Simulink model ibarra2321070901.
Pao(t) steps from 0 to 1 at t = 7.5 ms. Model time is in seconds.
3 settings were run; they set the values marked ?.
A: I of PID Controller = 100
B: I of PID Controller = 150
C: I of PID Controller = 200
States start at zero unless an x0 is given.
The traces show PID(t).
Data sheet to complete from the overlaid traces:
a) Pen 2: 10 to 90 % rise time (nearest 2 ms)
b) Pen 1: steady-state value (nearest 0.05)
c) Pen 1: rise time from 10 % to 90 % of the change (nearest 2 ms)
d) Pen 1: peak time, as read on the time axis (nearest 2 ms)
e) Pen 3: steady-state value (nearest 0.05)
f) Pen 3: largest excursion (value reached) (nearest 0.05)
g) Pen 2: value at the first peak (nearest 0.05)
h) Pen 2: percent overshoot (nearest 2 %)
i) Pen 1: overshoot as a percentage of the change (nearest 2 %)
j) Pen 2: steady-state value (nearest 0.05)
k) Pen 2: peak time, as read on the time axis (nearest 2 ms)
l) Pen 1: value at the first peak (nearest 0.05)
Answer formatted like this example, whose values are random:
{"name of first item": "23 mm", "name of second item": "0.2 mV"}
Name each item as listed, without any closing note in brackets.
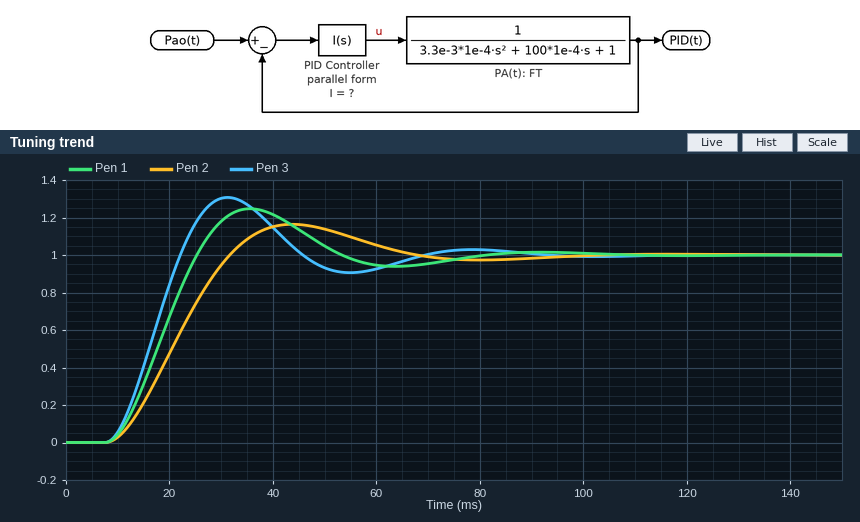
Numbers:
{"Pen 2: 10 to 90 % rise time": "16 ms", "Pen 1: steady-state value": "1.00", "Pen 1: rise time from 10 % to 90 % of the change": "12 ms", "Pen 1: peak time, as read on the time axis": "36 ms", "Pen 3: steady-state value": "1.00", "Pen 3: largest excursion (value reached)": "1.30", "Pen 2: value at the first peak": "1.15", "Pen 2: percent overshoot": "16 %", "Pen 1: overshoot as a percentage of the change": "24 %", "Pen 2: steady-state value": "1.00", "Pen 2: peak time, as read on the time axis": "44 ms", "Pen 1: value at the first peak": "1.25"}
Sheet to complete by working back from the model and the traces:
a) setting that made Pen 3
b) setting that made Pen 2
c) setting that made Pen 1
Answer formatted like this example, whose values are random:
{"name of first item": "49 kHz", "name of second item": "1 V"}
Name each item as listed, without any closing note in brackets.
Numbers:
{"setting that made Pen 3": "C", "setting that made Pen 2": "A", "setting that made Pen 1": "B"}
